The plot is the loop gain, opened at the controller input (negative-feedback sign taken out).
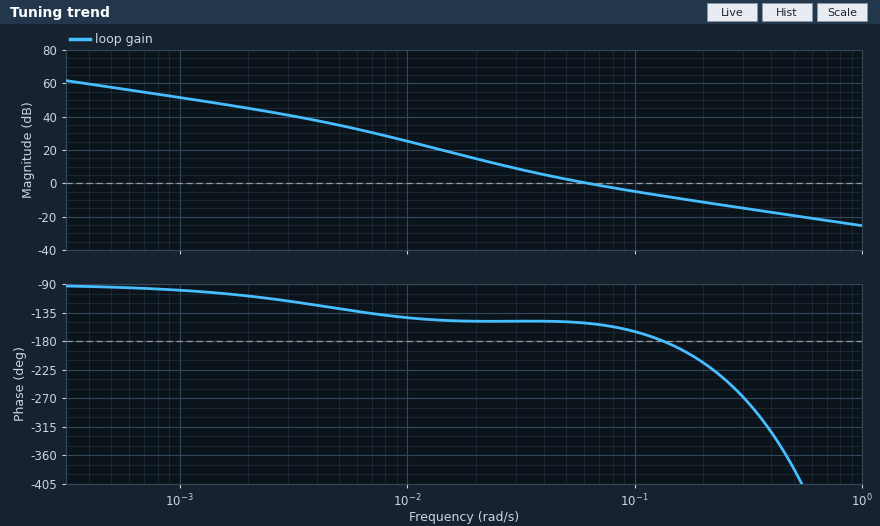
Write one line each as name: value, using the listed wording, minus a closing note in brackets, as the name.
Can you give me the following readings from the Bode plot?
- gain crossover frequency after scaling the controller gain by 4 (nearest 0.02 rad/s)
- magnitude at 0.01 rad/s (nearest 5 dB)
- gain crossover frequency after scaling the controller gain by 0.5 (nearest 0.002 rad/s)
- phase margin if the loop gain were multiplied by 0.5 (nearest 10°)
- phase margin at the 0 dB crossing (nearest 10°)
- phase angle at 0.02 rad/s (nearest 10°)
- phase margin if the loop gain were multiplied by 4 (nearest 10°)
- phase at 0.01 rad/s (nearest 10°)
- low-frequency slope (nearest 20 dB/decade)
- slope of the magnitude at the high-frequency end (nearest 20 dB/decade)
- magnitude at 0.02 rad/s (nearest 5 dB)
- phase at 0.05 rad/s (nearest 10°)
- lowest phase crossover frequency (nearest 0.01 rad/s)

gain crossover frequency after scaling the controller gain by 4: 0.22 rad/s
magnitude at 0.01 rad/s: 25 dB
gain crossover frequency after scaling the controller gain by 0.5: 0.038 rad/s
phase margin if the loop gain were multiplied by 0.5: 30°
phase margin at the 0 dB crossing: 30°
phase angle at 0.02 rad/s: -150°
phase margin if the loop gain were multiplied by 4: -40°
phase at 0.01 rad/s: -140°
low-frequency slope: -20 dB/decade
slope of the magnitude at the high-frequency end: -20 dB/decade
magnitude at 0.02 rad/s: 15 dB
phase at 0.05 rad/s: -150°
lowest phase crossover frequency: 0.13 rad/s
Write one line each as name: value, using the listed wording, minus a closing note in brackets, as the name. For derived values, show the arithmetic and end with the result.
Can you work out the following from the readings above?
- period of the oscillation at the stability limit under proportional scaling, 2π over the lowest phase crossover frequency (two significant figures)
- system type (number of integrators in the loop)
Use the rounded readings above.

period of the oscillation at the stability limit under proportional scaling, 2π over the lowest phase crossover frequency: 2π / 0.13 = 48 s
system type: 1
